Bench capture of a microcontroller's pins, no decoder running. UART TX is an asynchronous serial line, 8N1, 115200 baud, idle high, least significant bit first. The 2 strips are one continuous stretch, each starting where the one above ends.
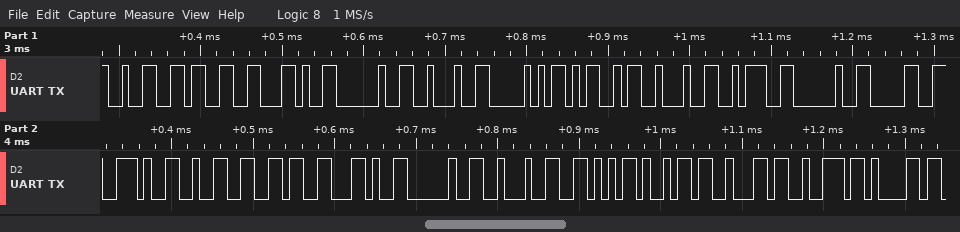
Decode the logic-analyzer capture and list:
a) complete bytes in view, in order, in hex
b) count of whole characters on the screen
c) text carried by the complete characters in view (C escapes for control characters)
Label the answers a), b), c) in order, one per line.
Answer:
a) 32 33 2C 20 22 50 4D 22 3A 20 30 2E 32 36 2C 20 22 56 69 62 72 61
b) 22
c) "23, \"PM\": 0.26, \"Vibra"
